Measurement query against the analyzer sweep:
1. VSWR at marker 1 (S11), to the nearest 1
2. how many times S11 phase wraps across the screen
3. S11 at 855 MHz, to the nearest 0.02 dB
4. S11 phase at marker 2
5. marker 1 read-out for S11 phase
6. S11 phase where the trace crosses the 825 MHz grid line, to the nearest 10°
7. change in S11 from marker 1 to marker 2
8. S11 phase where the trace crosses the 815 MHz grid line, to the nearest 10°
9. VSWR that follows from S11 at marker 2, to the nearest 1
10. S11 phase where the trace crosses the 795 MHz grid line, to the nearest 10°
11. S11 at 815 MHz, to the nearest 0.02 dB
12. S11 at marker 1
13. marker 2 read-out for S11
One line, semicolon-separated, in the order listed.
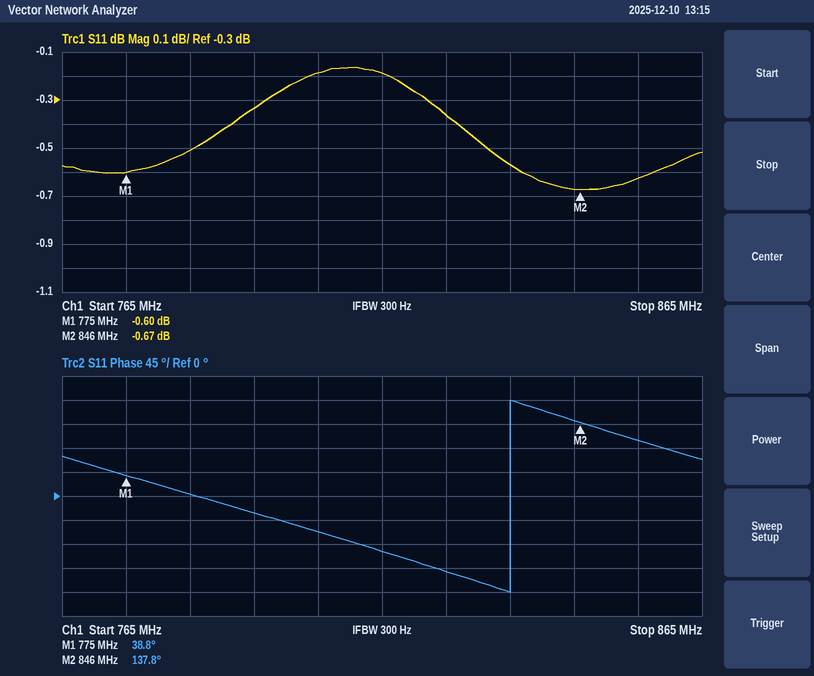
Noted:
29; 1; -0.62 dB; 137.8°; 38.8°; -140°; -0.07 dB; -100°; 26; -30°; -0.18 dB; -0.60 dB; -0.67 dB
